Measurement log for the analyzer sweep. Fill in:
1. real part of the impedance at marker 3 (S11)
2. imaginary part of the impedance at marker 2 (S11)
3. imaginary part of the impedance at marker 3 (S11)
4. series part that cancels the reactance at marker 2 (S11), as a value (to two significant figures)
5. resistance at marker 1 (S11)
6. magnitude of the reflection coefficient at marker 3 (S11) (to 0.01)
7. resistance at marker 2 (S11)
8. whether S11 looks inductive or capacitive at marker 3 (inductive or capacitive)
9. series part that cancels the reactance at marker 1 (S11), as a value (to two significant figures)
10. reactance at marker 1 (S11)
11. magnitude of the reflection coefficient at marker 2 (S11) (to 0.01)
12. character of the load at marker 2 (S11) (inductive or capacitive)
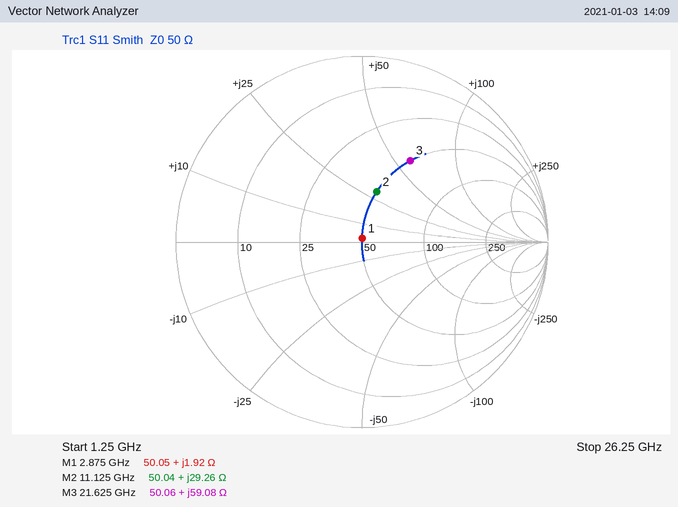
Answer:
50.06 Ω
+29.26 Ω
+59.08 Ω
490 fF
50.05 Ω
0.51
50.04 Ω
inductive
29 pF
+1.92 Ω
0.28
inductive
